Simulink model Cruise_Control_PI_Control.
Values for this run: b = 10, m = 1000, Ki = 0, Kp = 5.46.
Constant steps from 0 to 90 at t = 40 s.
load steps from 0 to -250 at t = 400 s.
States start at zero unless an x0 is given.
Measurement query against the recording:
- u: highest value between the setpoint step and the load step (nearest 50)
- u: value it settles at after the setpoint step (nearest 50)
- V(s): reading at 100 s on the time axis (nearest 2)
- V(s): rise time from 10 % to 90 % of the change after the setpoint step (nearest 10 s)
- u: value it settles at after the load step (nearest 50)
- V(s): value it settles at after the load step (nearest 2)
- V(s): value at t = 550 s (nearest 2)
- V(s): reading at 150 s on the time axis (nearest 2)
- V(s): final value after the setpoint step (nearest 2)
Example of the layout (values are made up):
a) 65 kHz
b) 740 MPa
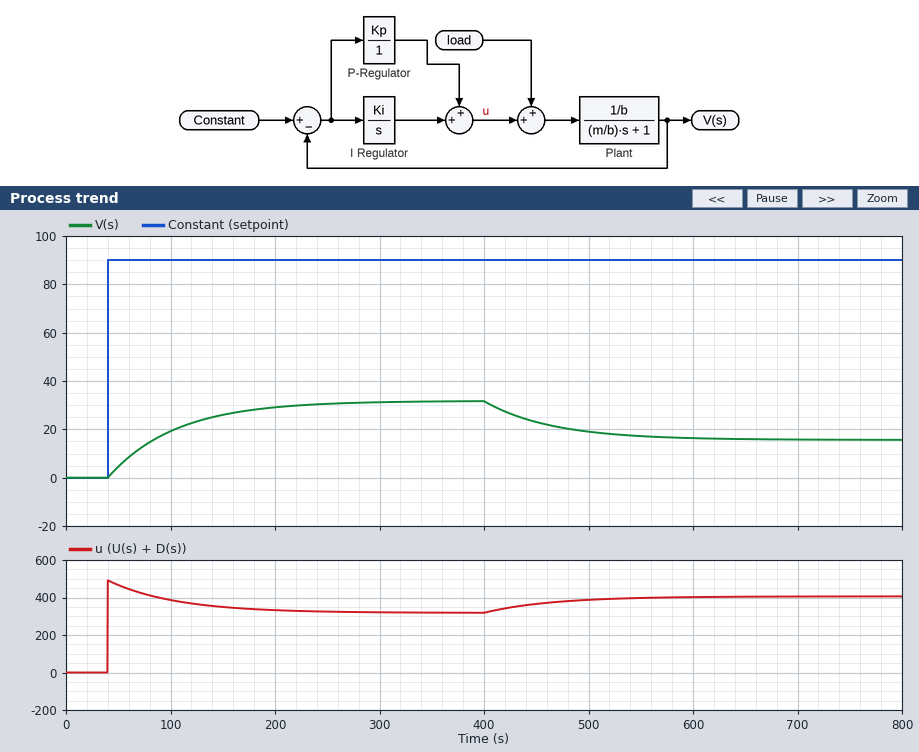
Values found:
a) 500
b) 300
c) 20
d) 140 s
e) 400
f) 16
g) 18
h) 26
i) 32
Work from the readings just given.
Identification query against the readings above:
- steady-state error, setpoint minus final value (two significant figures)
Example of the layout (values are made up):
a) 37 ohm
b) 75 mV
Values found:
a) 58
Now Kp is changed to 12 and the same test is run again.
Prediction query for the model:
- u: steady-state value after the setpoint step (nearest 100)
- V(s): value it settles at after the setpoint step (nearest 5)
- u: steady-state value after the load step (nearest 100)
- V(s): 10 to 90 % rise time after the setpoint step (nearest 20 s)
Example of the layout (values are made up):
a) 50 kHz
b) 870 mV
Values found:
a) 500
b) 50
c) 600
d) 100 s
